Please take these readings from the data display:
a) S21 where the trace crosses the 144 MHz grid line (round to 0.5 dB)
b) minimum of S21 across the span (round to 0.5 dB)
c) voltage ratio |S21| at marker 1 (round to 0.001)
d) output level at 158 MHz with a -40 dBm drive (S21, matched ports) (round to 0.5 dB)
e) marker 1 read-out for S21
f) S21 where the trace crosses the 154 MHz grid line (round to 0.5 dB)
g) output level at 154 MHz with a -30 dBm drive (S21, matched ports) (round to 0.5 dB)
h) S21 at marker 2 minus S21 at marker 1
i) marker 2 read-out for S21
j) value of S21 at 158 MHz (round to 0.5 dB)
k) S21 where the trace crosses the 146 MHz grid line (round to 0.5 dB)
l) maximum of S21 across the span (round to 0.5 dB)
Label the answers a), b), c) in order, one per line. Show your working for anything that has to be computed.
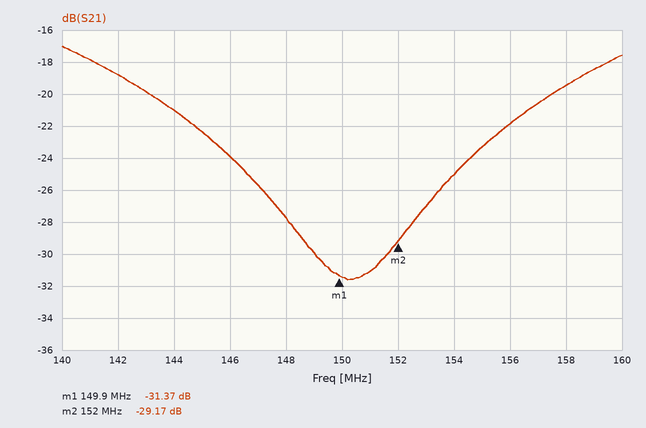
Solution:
a) -21.0 dB
b) -31.5 dB
c) 10^(-31.37/20) ≈ 0.027
d) -40 dBm + (-19.5 dB) = -59.5 dBm
e) -31.37 dB
f) -25.0 dB
g) -30 dBm + (-25.0 dB) = -55.0 dBm
h) -29.17 − (-31.37) = 2.20 dB
i) -29.17 dB
j) -19.5 dB
k) -24.0 dB
l) -17.0 dB
